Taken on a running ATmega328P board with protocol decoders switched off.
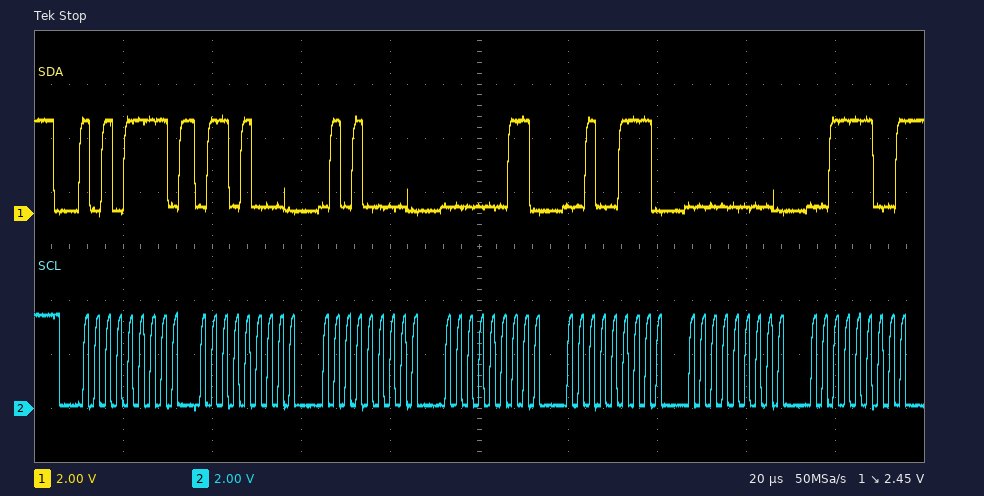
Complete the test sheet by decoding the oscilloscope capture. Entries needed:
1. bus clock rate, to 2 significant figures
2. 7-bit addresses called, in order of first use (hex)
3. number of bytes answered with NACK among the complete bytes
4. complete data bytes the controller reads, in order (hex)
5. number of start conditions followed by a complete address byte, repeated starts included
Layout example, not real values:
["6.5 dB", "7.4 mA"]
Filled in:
["400 kHz", "0x57", "1", "68 50 03 27 00 3C", "1"]
